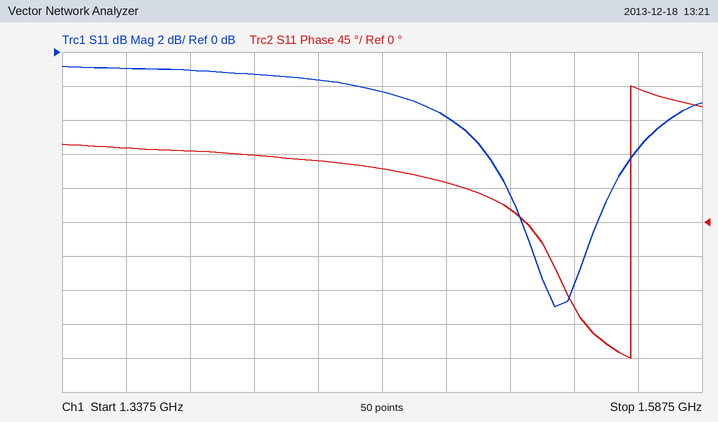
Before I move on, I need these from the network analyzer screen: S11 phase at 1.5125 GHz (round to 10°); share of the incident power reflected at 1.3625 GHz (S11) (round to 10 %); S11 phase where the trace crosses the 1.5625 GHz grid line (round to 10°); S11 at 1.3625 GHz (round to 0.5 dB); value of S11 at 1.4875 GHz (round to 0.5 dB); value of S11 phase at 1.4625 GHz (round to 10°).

20°
80 %
180°
-1.0 dB
-4.0 dB
70°
